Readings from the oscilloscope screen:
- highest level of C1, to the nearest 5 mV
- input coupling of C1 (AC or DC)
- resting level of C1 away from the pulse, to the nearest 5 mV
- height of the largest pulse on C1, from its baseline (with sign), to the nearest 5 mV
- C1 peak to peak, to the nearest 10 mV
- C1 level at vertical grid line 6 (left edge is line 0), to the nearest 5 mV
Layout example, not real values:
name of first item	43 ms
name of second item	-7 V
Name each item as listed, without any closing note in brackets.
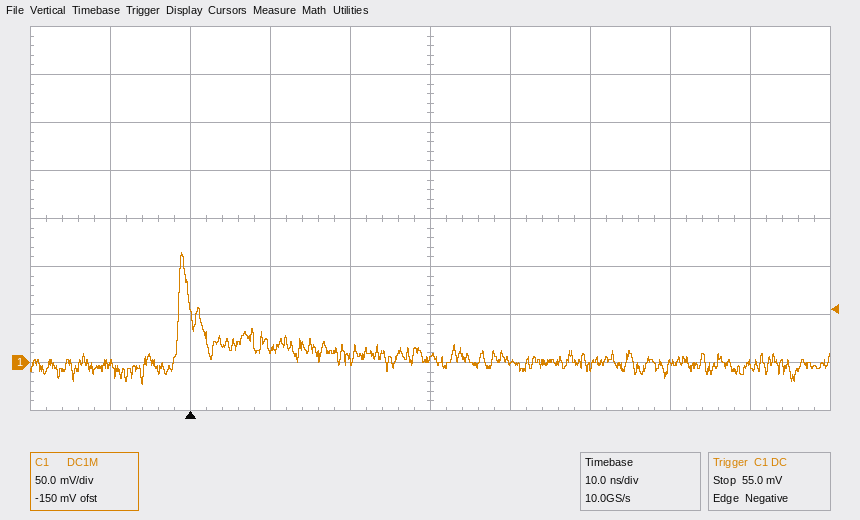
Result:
highest level of C1, to the nearest 5 mV	115 mV
input coupling of C1	DC
resting level of C1 away from the pulse, to the nearest 5 mV	0 mV
height of the largest pulse on C1, from its baseline (with sign), to the nearest 5 mV	+115 mV
C1 peak to peak, to the nearest 10 mV	140 mV
C1 level at vertical grid line 6 (left edge is line 0), to the nearest 5 mV	0 mV
